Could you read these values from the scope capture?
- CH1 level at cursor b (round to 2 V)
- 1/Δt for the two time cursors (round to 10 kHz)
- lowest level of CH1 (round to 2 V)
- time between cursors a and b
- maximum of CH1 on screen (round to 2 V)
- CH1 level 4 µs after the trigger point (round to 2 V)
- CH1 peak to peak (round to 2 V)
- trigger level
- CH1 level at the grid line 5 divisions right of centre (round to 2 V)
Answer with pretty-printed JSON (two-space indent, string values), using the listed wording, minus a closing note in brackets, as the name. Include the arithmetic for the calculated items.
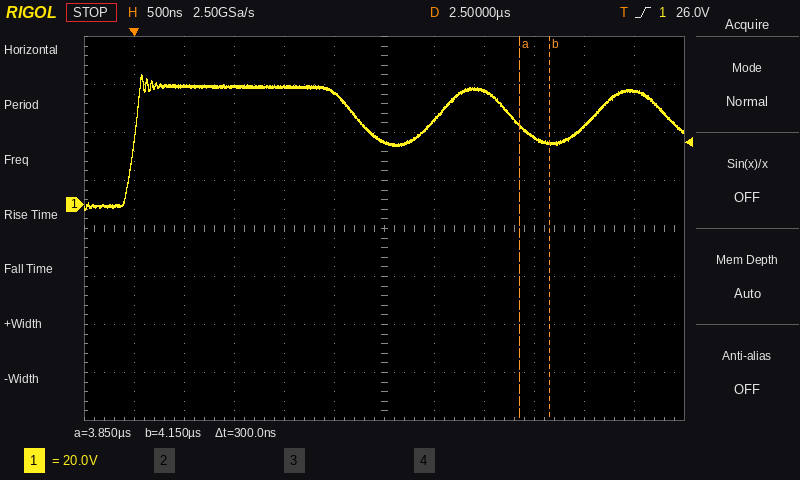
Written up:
{
  "CH1 level at cursor b": "26 V",
  "1/Δt for the two time cursors": "1 / 300 ns ≈ 3.33 MHz",
  "lowest level of CH1": "-2 V",
  "time between cursors a and b": "300 ns",
  "maximum of CH1 on screen": "54 V",
  "CH1 level 4 µs after the trigger point": "28 V",
  "CH1 peak to peak": "54 V − (-2 V) = 56 V",
  "trigger level": "26.0 V",
  "CH1 level at the grid line 5 divisions right of centre": "48 V"
}
